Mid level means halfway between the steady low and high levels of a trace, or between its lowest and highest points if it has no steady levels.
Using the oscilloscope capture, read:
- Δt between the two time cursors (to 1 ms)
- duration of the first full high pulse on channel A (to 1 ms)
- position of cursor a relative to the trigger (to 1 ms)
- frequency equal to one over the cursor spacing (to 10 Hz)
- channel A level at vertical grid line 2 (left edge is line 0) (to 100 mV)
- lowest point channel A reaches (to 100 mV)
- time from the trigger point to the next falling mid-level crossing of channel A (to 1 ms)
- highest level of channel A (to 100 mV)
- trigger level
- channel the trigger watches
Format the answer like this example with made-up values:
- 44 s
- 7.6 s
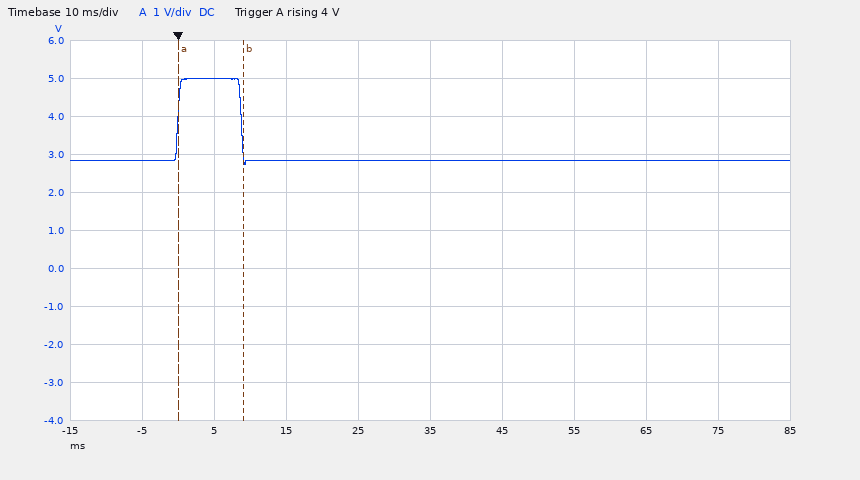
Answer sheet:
- 9 ms
- 9 ms
- 0 ms
- 110 Hz
- 5.0 V
- 2.7 V
- 9 ms
- 5.0 V
- 4 V
- channel A
